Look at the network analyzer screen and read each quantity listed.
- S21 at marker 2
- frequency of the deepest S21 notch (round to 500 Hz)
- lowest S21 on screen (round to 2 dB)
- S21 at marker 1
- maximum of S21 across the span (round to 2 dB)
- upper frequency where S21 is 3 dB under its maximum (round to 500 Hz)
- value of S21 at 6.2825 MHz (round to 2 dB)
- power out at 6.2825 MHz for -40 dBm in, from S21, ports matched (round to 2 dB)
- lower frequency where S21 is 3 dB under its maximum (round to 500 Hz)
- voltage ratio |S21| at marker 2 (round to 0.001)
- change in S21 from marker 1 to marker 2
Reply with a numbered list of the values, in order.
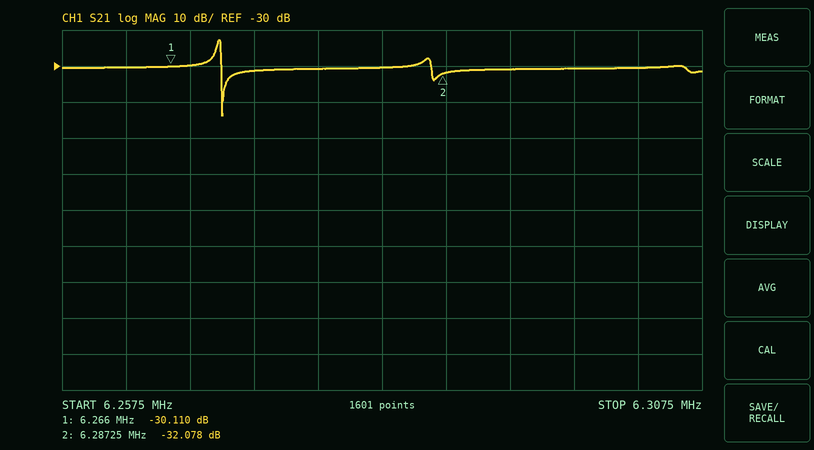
1. -32.078 dB
2. 6.2700 MHz
3. -44 dB
4. -30.110 dB
5. -22 dB
6. 6.2700 MHz
7. -30 dB
8. -70 dBm
9. 6.2695 MHz
10. 0.025
11. -1.968 dB
